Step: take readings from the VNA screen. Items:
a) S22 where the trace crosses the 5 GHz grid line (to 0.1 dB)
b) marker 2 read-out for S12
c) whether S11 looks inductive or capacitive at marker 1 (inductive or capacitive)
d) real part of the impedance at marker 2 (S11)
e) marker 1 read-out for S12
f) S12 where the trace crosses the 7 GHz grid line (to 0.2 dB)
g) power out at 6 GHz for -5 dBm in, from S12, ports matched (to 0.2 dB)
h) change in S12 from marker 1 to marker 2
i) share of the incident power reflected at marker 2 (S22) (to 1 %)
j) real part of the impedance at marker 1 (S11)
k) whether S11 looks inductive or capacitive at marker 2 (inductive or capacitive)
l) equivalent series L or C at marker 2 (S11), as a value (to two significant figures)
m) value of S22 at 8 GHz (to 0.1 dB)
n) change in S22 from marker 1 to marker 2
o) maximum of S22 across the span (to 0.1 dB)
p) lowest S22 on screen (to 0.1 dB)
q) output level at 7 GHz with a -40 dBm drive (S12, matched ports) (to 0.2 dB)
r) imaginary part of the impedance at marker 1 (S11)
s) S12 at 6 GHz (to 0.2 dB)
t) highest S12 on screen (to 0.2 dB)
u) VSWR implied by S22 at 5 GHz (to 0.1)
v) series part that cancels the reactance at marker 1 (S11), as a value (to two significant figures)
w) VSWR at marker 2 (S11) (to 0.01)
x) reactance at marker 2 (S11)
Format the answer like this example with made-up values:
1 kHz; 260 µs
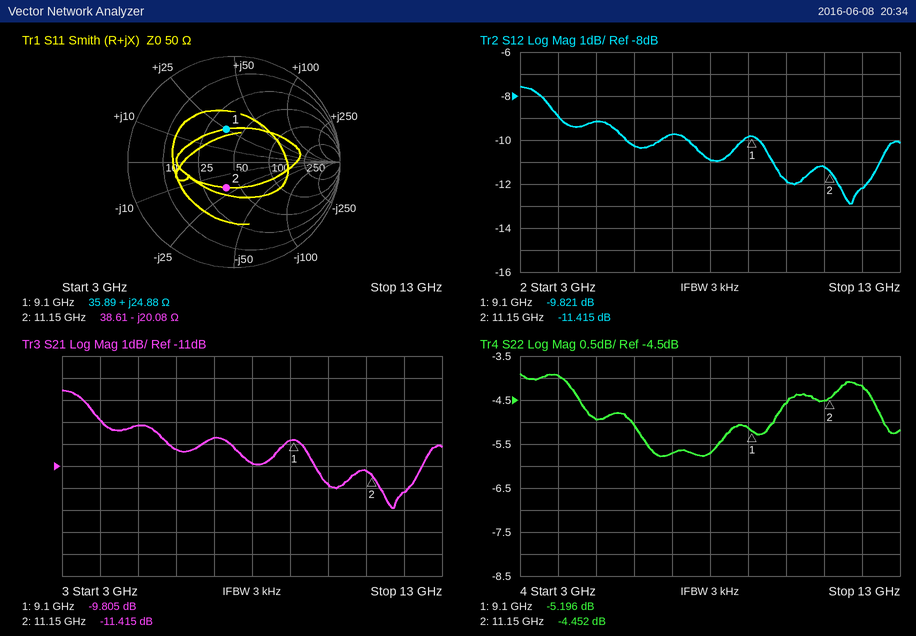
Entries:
-4.9 dB; -11.415 dB; inductive; 38.61 Ω; -9.821 dB; -9.8 dB; -15.2 dBm; -1.594 dB; 36 %; 35.89 Ω; capacitive; 710 fF; -5.7 dB; 0.744 dB; -3.9 dB; -5.8 dB; -49.8 dBm; +24.88 Ω; -10.2 dB; -7.6 dB; 3.6; 700 fF; 1.68; -20.08 Ω
